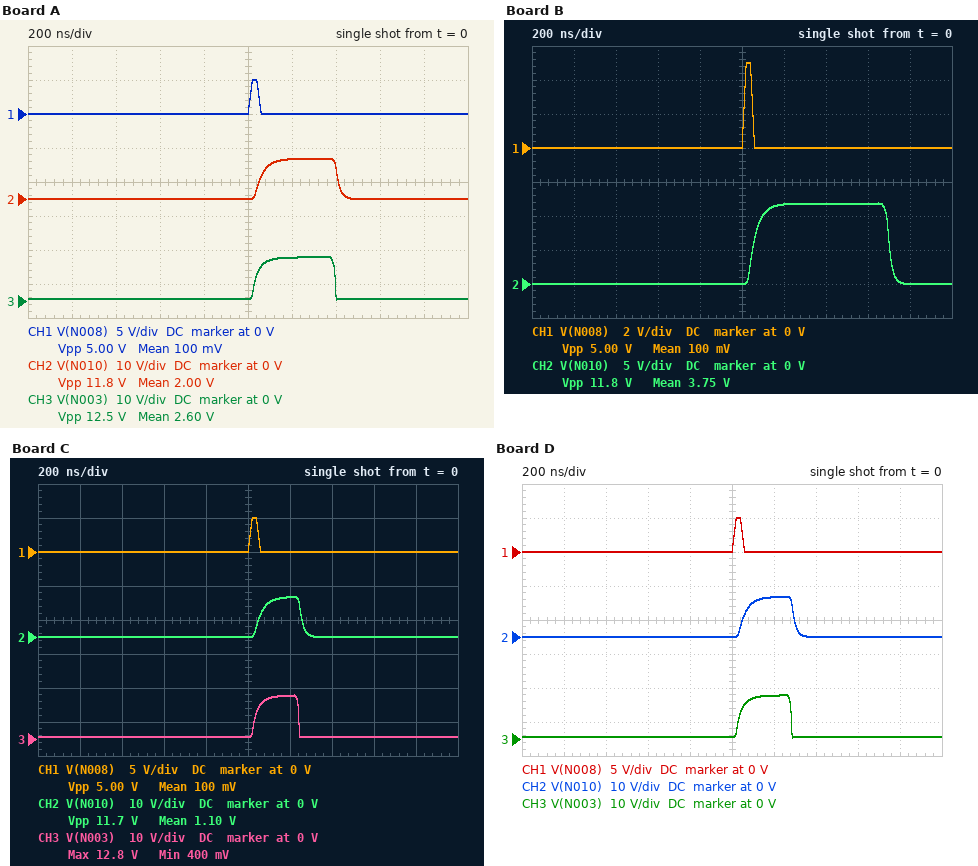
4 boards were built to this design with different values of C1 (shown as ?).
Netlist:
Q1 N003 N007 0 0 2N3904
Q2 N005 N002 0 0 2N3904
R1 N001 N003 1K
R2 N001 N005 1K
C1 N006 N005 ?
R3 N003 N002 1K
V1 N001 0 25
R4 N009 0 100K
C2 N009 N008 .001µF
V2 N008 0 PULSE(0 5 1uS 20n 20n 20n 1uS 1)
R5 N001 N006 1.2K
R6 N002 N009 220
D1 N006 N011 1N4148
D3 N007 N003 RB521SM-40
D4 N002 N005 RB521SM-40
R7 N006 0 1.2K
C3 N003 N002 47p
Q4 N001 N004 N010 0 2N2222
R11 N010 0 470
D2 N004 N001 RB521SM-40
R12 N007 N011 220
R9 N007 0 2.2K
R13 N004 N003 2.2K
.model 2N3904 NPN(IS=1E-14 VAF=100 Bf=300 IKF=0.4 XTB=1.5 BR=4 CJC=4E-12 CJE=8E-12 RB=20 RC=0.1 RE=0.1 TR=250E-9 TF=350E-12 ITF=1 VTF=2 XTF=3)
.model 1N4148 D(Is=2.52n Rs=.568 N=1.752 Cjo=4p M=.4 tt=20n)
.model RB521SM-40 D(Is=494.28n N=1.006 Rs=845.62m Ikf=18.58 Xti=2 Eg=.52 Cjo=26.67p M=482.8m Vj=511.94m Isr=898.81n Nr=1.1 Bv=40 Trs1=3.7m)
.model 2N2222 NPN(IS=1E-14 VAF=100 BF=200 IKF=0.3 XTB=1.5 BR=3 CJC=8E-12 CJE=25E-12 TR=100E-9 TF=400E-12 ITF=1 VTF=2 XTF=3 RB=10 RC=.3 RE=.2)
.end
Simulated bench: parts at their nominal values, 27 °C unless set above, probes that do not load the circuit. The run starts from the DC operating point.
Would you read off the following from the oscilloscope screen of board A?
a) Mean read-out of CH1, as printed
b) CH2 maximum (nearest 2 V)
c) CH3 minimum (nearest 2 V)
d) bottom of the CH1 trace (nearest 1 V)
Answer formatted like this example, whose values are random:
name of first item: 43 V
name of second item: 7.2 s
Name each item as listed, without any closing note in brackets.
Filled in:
Mean read-out of CH1, as printed: 100 mV
CH2 maximum: 12 V
CH3 minimum: 0 V
bottom of the CH1 trace: 0 V
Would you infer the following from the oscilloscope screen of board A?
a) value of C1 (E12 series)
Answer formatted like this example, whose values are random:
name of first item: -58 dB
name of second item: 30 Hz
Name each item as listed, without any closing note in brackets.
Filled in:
value of C1: 560 pF
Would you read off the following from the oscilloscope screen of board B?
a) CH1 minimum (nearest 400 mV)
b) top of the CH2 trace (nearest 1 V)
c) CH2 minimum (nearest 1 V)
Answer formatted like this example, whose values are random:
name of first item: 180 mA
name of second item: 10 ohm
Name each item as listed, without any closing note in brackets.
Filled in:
CH1 minimum: 0 V
top of the CH2 trace: 12 V
CH2 minimum: 0 V
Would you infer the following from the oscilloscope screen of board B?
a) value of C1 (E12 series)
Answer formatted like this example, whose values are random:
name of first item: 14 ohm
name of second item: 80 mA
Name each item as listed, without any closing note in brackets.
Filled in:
value of C1: 1 nF
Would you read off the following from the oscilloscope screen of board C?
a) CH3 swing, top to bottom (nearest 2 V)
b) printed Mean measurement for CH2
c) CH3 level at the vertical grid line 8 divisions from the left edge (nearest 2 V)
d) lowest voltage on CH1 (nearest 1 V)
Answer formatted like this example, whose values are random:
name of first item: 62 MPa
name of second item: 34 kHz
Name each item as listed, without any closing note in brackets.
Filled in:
CH3 swing, top to bottom: 12 V
printed Mean measurement for CH2: 1.10 V
CH3 level at the vertical grid line 8 divisions from the left edge: 0 V
lowest voltage on CH1: 0 V
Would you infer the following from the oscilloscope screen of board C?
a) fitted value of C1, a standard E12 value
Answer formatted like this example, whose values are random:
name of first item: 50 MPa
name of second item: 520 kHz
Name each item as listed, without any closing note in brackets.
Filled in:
fitted value of C1, a standard E12 value: 330 pF
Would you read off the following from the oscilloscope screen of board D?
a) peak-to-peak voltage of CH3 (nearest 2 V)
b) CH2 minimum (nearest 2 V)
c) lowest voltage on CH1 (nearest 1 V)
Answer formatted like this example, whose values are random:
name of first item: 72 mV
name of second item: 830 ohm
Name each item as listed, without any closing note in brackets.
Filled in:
peak-to-peak voltage of CH3: 12 V
CH2 minimum: 0 V
lowest voltage on CH1: 0 V
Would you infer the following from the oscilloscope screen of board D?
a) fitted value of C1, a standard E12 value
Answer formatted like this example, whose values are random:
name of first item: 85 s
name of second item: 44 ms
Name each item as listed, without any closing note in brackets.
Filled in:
fitted value of C1, a standard E12 value: 390 pF
